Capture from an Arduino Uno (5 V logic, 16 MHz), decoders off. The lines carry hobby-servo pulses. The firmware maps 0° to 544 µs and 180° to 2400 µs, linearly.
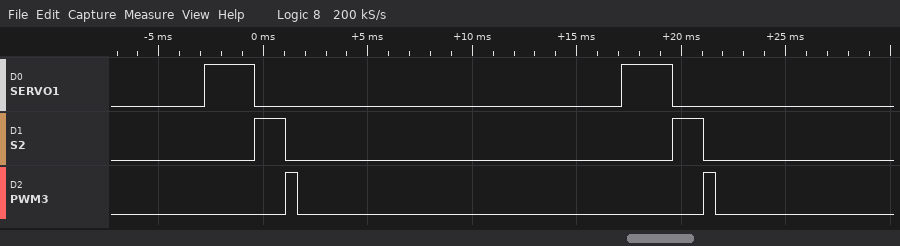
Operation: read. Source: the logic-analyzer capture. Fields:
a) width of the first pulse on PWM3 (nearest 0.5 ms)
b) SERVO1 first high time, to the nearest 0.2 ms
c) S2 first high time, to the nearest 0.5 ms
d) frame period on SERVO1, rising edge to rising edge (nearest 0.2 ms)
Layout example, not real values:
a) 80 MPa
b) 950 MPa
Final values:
a) 0.5 ms
b) 2.4 ms
c) 1.5 ms
d) 20.0 ms
